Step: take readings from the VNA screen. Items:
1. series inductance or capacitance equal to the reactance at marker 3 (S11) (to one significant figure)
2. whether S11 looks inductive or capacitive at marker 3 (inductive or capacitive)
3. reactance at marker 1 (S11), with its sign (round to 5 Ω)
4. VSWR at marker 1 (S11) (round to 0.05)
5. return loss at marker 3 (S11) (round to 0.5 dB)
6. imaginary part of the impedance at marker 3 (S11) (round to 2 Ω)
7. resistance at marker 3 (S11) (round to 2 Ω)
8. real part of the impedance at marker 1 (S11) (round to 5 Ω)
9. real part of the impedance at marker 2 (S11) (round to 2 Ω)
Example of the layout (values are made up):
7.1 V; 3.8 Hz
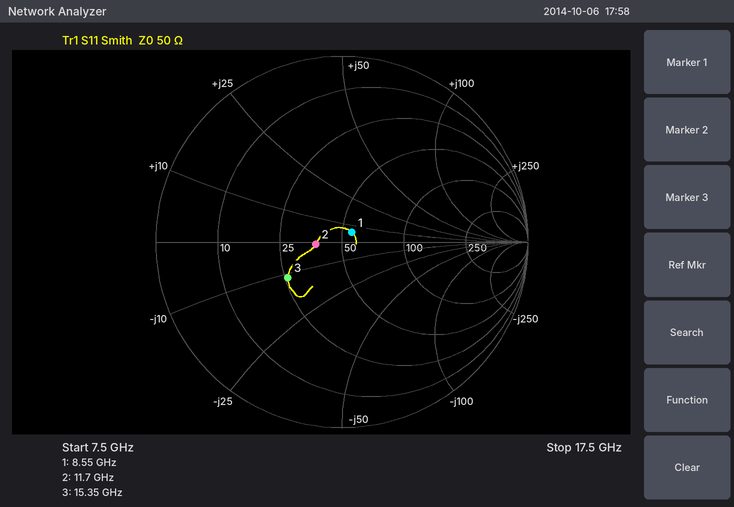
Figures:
900 fF; capacitive; +5 Ω; 1.15; 9.0 dB; -12 Ω; 26 Ω; 55 Ω; 38 Ω
